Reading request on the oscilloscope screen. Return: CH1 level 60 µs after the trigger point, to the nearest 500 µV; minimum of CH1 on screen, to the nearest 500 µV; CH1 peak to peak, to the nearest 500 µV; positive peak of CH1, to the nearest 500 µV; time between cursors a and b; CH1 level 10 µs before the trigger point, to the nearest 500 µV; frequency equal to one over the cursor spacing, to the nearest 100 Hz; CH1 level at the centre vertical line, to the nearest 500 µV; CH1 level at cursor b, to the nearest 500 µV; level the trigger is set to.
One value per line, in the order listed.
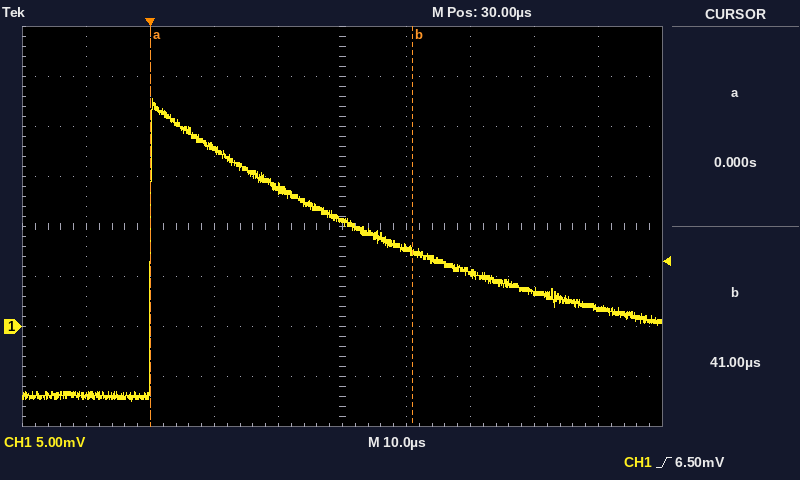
3.5 mV
-7.5 mV
30.5 mV
23.0 mV
41 µs
-7.0 mV
24.4 kHz
10.5 mV
7.5 mV
6.50 mV
